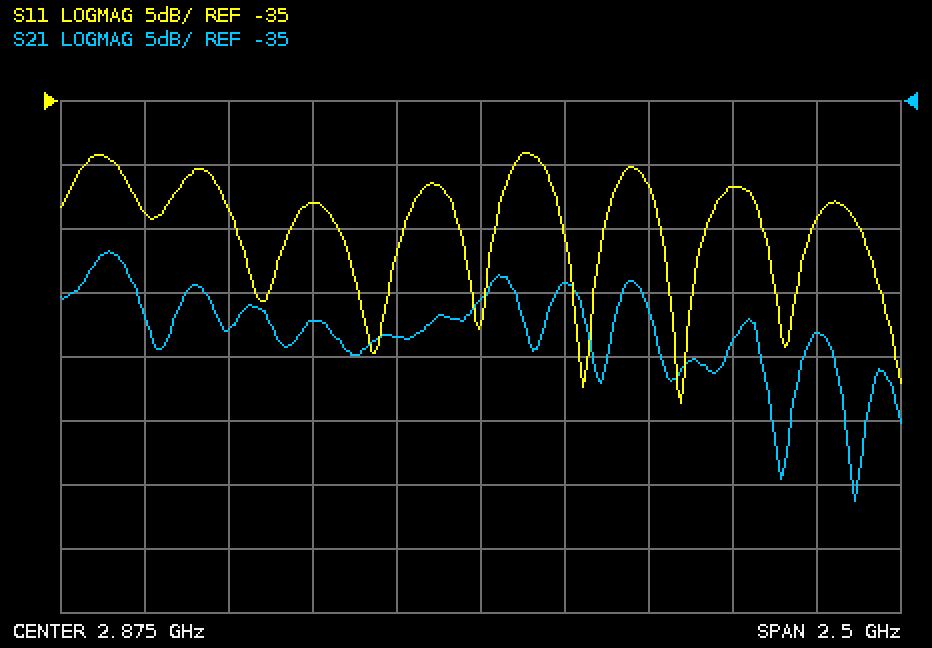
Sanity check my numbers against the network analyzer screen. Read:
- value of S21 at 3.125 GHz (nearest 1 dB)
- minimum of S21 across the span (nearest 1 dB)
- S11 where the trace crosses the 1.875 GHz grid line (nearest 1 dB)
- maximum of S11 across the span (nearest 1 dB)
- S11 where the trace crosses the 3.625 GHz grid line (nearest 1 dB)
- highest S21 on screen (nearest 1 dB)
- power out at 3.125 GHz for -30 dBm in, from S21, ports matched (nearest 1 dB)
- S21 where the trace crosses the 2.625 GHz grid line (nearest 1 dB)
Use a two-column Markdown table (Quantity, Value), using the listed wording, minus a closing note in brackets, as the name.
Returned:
| Quantity | Value |
|---|---|
| value of S21 at 3.125 GHz | -49 dB |
| minimum of S21 across the span | -66 dB |
| S11 where the trace crosses the 1.875 GHz grid line | -44 dB |
| maximum of S11 across the span | -39 dB |
| S11 where the trace crosses the 3.625 GHz grid line | -42 dB |
| highest S21 on screen | -47 dB |
| power out at 3.125 GHz for -30 dBm in, from S21, ports matched | -79 dBm |
| S21 where the trace crosses the 2.625 GHz grid line | -53 dB |
